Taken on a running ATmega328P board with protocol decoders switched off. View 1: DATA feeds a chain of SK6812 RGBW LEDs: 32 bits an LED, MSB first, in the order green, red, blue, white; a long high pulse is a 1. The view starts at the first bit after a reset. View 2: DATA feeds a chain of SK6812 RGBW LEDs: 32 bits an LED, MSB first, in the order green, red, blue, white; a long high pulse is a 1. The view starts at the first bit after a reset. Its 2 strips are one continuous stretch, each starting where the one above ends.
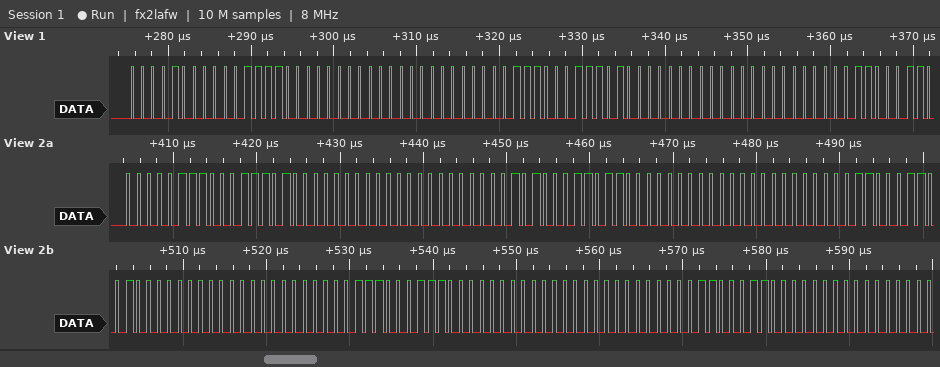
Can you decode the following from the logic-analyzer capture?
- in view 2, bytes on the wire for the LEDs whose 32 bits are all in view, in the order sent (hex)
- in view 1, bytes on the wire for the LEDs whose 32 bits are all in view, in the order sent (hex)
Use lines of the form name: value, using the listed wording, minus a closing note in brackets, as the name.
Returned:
in view 2, bytes on the wire for the LEDs whose 32 bits are all in view, in the order sent: 07 1D 00 00 05 1B 00 00 03 19 00 00 07 1C 00 00
in view 1, bytes on the wire for the LEDs whose 32 bits are all in view, in the order sent: 08 1E 00 00 07 1D 00 00
